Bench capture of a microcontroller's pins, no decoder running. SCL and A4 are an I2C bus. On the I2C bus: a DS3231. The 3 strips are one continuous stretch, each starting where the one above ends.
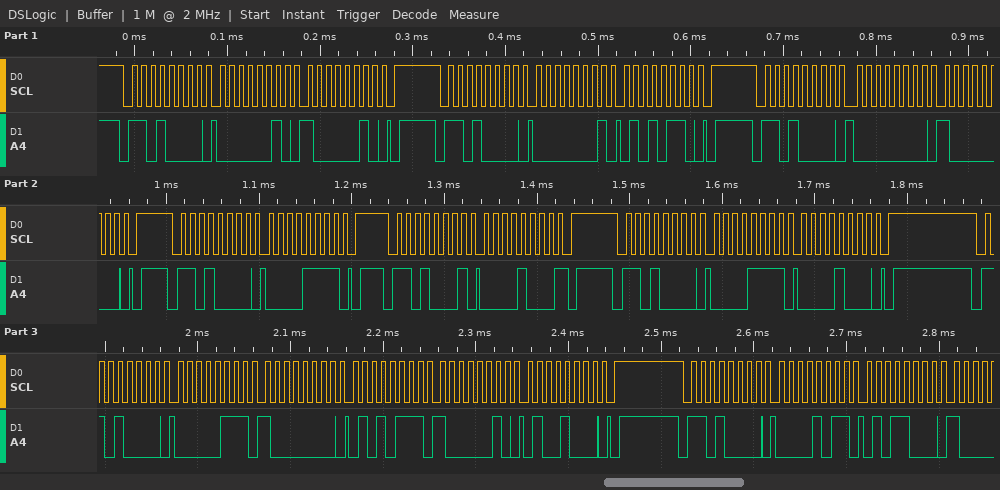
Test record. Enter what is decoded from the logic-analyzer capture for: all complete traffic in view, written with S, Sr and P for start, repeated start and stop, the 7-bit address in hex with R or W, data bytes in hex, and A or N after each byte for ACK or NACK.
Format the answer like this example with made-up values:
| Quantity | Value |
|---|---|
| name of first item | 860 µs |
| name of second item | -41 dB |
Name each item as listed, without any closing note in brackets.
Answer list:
| Quantity | Value |
|---|---|
| all complete traffic in view, written with S, Sr and P for start, repeated start and stop, the 7-bit address in hex with R or W, data bytes in hex, and A or N after each byte for ACK or NACK | S 68W A 02 A 82 A P S 68W A 01 A 56 A P S 68W A 00 A 80 A P S 68W A 0F A P S 68R A 08 N P S 68W A 0F A 08 A P S 68W A 07 A 80 A 57 A 82 A 48 A P S 68W A 0B A 58 A |
